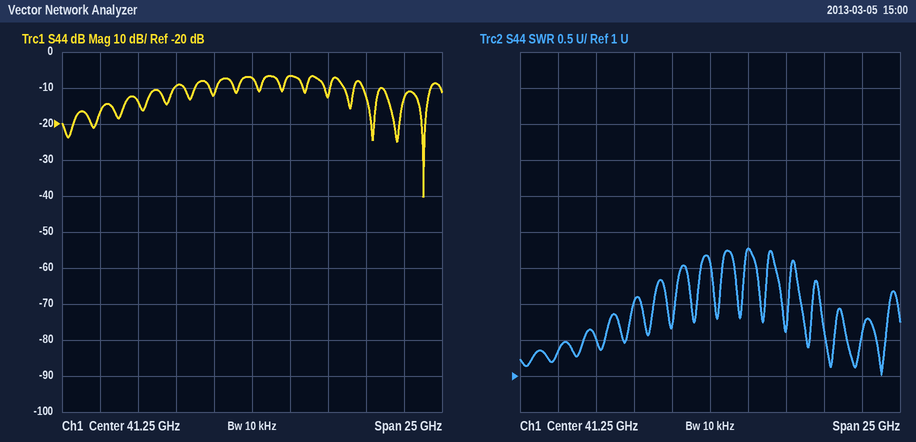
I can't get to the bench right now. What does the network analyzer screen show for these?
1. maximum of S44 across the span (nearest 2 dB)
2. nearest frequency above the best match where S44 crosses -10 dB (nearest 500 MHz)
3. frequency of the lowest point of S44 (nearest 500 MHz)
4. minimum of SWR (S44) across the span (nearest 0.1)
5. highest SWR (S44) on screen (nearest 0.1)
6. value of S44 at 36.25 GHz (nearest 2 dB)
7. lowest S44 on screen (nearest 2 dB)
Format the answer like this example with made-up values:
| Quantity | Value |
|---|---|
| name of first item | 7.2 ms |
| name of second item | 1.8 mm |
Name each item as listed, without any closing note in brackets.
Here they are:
| Quantity | Value |
|---|---|
| maximum of S44 across the span | -6 dB |
| nearest frequency above the best match where S44 crosses -10 dB | 53.0 GHz |
| frequency of the lowest point of S44 | 52.5 GHz |
| minimum of SWR (S44) across the span | 1.0 |
| highest SWR (S44) on screen | 2.8 |
| value of S44 at 36.25 GHz | -10 dB |
| lowest S44 on screen | -40 dB |
